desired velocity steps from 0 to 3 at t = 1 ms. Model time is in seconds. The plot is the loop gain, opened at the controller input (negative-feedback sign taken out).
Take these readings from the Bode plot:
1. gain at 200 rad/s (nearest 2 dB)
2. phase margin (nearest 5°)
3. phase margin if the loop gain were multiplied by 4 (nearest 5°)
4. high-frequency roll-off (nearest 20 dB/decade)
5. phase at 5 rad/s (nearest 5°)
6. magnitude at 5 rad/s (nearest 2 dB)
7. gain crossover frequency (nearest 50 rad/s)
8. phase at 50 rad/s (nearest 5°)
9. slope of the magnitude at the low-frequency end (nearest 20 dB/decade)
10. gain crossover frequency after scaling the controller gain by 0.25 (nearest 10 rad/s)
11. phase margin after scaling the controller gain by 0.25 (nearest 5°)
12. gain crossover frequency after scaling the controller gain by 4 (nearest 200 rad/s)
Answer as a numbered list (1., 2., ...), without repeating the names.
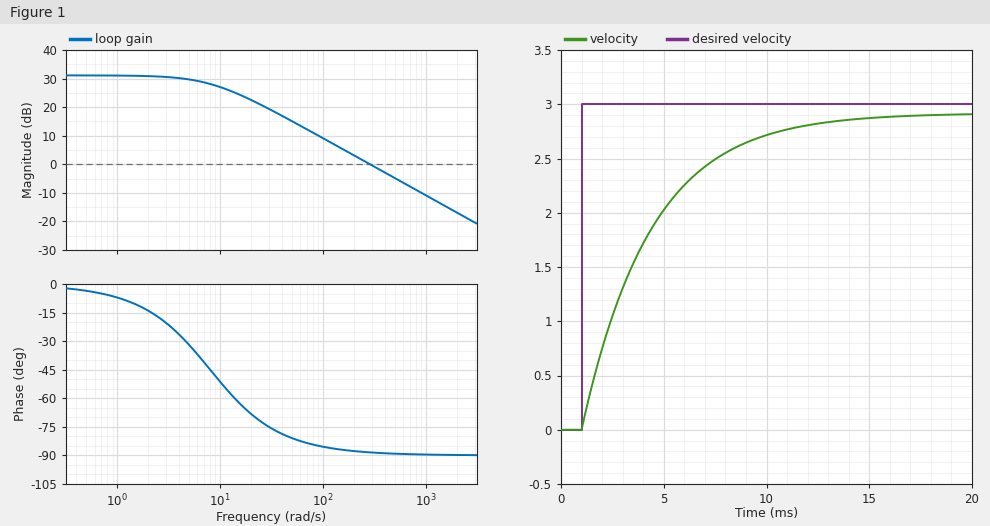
1. 4 dB
2. 90°
3. 90°
4. -20 dB/decade
5. -30°
6. 30 dB
7. 300 rad/s
8. -80°
9. 0 dB/decade
10. 70 rad/s
11. 95°
12. 1200 rad/s
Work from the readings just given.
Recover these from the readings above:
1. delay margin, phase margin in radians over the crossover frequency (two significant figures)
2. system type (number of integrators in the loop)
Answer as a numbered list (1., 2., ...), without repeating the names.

1. 0.0052 s
2. 0
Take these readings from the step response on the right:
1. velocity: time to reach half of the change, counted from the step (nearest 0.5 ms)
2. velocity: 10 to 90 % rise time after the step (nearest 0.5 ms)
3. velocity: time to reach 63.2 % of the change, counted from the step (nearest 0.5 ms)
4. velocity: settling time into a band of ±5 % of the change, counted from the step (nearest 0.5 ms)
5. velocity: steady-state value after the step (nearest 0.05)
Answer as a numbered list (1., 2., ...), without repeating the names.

1. 2.5 ms
2. 7.5 ms
3. 3.5 ms
4. 10.0 ms
5. 2.90
